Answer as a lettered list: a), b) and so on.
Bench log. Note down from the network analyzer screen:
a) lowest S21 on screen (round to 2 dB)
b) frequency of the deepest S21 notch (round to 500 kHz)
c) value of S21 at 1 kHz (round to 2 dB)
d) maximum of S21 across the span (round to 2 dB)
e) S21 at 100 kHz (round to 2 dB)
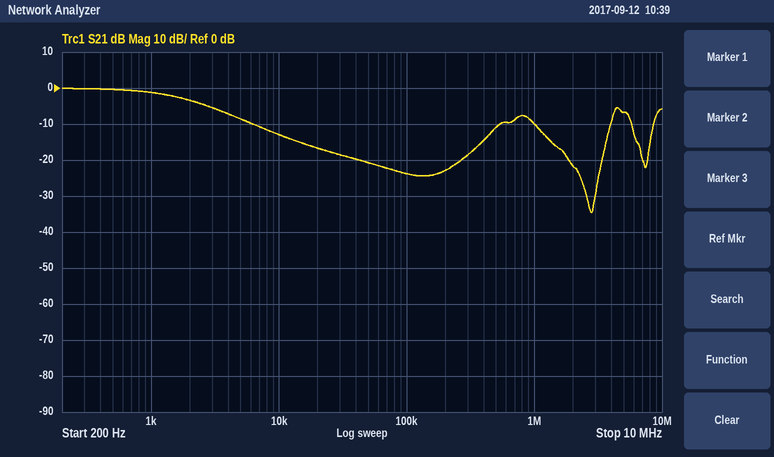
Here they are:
a) -34 dB
b) 3.0 MHz
c) -2 dB
d) 0 dB
e) -24 dB
